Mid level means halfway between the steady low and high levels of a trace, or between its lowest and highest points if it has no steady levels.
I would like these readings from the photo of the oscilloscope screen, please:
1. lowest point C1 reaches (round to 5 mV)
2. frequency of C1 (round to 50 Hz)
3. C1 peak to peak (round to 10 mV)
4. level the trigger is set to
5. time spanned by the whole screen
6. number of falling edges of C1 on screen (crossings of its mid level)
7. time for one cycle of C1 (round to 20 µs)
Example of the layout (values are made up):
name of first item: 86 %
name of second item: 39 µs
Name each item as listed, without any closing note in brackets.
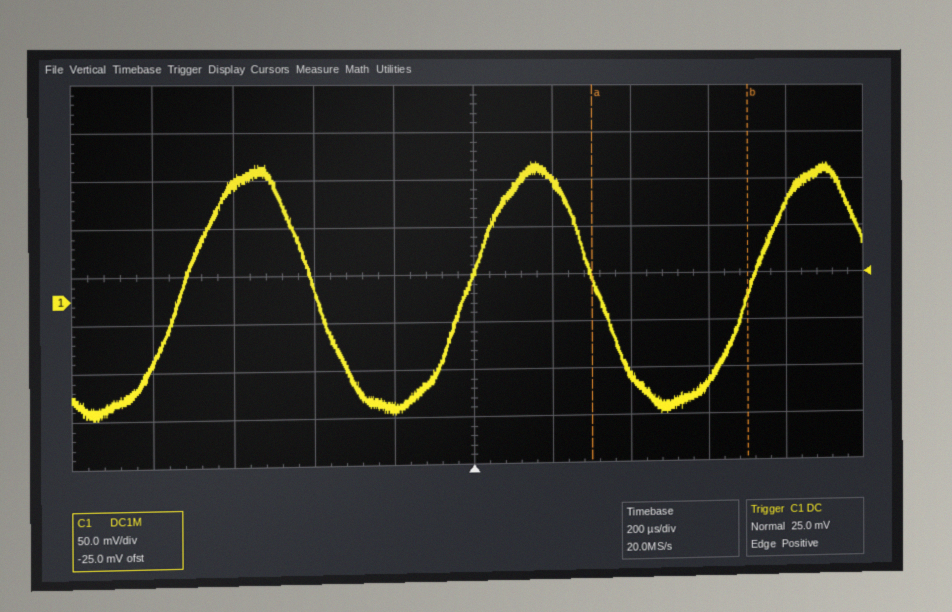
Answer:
lowest point C1 reaches: -125 mV
frequency of C1: 1.40 kHz
C1 peak to peak: 270 mV
level the trigger is set to: 25.0 mV
time spanned by the whole screen: 2 ms
number of falling edges of C1 on screen: 2
time for one cycle of C1: 720 µs
